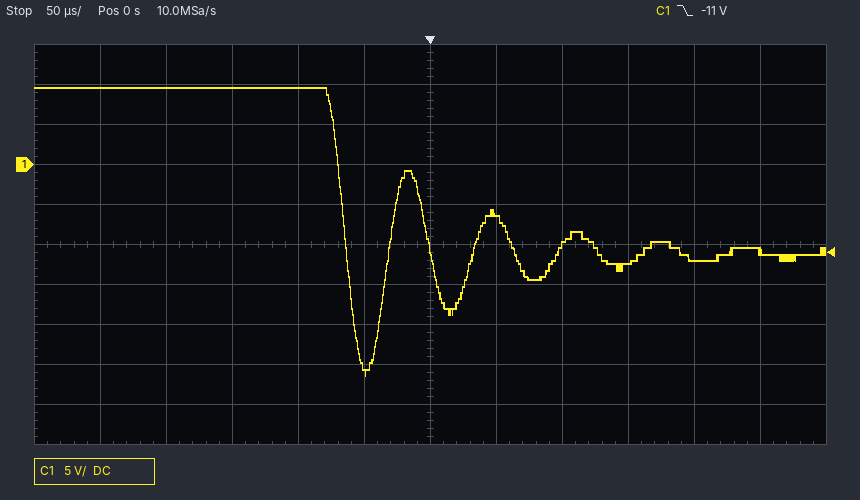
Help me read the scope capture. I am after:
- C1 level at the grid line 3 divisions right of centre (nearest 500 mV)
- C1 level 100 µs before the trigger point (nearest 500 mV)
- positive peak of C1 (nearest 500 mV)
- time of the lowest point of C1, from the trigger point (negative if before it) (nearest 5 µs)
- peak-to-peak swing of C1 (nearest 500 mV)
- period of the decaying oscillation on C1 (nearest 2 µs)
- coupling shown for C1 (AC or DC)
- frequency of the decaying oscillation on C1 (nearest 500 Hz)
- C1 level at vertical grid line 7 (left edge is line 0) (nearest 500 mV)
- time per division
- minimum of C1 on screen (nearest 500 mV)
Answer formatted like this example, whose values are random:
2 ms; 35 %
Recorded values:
-12.0 V; 9.5 V; 9.5 V; -50 µs; 36.0 V; 64 µs; DC; 15.5 kHz; -6.0 V; 50 µs; -26.5 V
